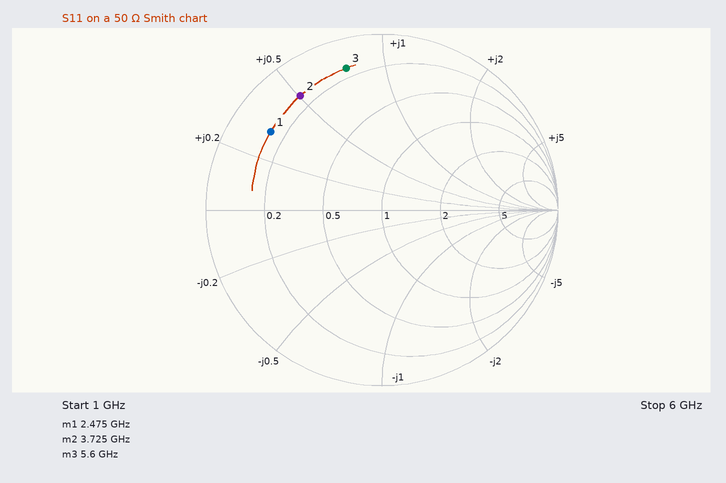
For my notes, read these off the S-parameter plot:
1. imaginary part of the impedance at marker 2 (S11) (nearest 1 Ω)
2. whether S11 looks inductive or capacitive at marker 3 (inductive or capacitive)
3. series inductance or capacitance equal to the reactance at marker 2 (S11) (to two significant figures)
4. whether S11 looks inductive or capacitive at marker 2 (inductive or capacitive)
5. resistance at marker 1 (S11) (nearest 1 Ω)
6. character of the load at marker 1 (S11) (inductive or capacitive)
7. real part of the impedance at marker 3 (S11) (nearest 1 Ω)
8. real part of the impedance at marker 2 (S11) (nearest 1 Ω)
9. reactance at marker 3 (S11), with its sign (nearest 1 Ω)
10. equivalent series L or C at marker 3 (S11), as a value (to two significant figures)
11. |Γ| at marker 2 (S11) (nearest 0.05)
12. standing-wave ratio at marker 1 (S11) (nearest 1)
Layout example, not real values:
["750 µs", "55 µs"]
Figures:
["+25 Ω", "inductive", "1.1 nH", "inductive", "7 Ω", "inductive", "7 Ω", "7 Ω", "+38 Ω", "1.1 nH", "0.80", "8"]
